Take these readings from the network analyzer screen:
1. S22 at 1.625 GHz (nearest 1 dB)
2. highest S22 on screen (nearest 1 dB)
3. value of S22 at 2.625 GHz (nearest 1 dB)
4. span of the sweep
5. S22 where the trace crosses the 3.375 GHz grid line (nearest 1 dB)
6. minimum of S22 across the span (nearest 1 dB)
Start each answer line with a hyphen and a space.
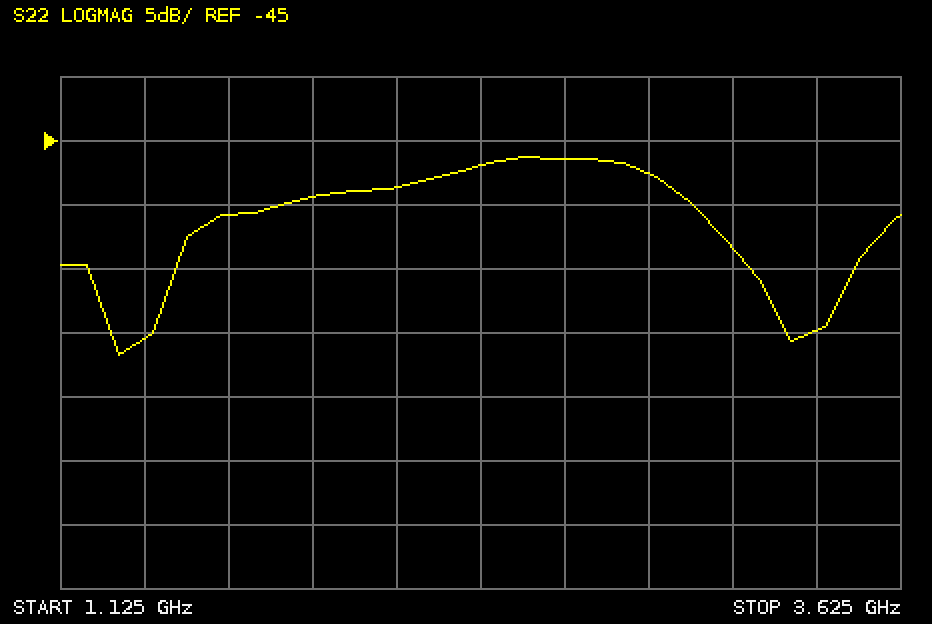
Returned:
- -51 dB
- -46 dB
- -46 dB
- 2.5 GHz
- -60 dB
- -62 dB
